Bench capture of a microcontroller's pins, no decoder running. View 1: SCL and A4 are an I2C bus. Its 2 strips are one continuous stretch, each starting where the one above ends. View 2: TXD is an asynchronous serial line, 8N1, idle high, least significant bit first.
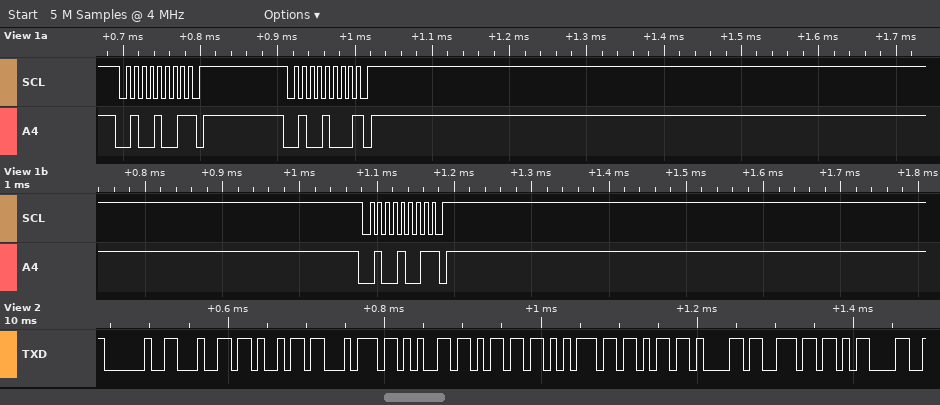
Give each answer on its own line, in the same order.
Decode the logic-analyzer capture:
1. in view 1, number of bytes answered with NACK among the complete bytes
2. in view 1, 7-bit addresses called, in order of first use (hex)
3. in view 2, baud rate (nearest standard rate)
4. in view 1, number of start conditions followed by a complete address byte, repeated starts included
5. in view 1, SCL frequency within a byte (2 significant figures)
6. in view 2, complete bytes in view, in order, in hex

3
0x24
115200 baud
3
100 kHz
0x20 0x64 0x69 0x74 0x65 0x6D 0x75 0x6B 0x61 0x6E 0x0D
